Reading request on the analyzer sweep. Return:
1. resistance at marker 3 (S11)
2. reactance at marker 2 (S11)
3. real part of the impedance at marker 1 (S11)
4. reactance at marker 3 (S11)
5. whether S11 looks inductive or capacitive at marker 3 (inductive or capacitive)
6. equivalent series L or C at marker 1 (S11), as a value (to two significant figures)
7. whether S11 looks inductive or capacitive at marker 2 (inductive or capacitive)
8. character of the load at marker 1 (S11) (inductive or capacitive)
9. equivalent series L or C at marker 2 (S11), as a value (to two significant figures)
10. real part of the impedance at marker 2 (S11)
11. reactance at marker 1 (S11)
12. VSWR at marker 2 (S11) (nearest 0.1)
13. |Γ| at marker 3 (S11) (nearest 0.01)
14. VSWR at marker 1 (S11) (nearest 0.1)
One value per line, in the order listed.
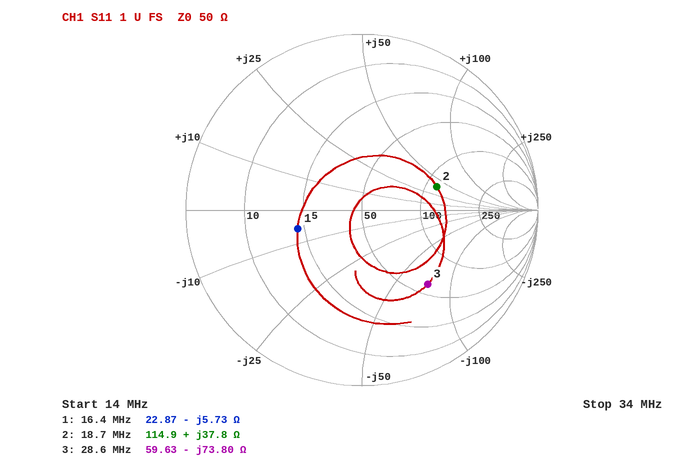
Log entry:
59.63 Ω
+37.8 Ω
22.87 Ω
-73.80 Ω
capacitive
1.7 nF
inductive
capacitive
320 nH
114.9 Ω
-5.73 Ω
2.6
0.56
2.2
